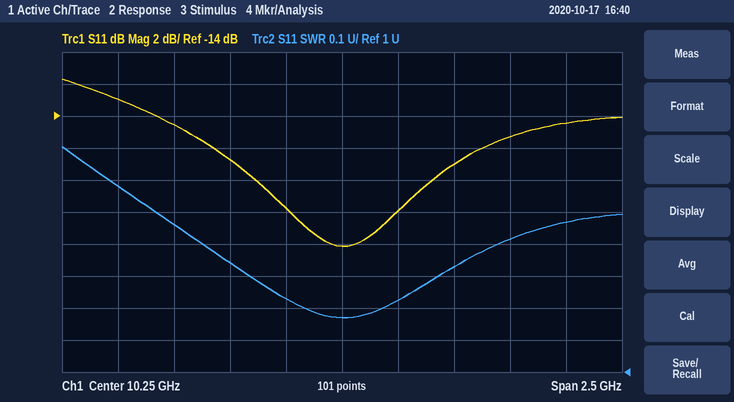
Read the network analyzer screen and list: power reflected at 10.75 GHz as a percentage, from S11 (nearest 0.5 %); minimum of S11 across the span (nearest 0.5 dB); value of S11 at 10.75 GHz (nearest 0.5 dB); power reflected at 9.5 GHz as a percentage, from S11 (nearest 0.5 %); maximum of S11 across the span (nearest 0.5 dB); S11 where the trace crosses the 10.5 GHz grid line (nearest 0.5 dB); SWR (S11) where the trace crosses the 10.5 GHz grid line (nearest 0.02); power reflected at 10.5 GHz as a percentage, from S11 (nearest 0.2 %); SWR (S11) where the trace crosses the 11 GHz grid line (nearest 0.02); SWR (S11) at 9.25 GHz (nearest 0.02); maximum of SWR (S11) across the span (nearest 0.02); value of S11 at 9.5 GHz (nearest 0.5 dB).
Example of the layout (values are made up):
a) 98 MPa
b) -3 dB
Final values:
a) 2.0 %
b) -22.0 dB
c) -17.0 dB
d) 3.5 %
e) -11.5 dB
f) -20.0 dB
g) 1.22
h) 1.0 %
i) 1.42
j) 1.58
k) 1.70
l) -14.5 dB
